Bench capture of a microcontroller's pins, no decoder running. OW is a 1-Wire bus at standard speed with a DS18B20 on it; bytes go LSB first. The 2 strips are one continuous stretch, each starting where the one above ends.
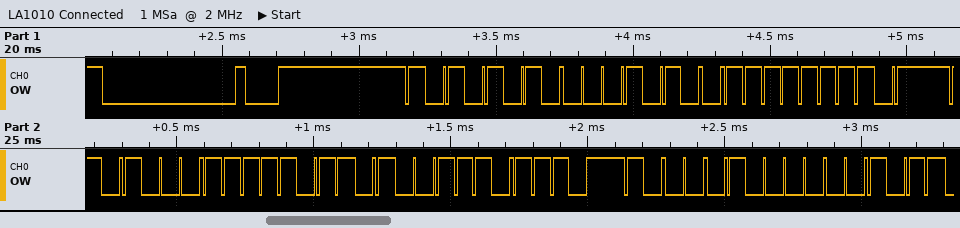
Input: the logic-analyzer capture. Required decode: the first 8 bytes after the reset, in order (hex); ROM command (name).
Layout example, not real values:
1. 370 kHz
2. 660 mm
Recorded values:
1. 55 28 FF 16 DF 72 17 02
2. Match ROM
